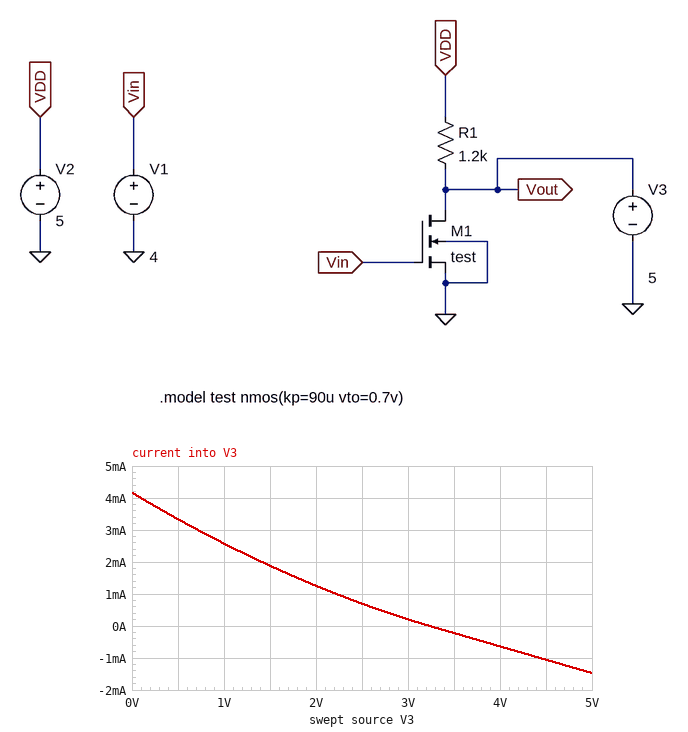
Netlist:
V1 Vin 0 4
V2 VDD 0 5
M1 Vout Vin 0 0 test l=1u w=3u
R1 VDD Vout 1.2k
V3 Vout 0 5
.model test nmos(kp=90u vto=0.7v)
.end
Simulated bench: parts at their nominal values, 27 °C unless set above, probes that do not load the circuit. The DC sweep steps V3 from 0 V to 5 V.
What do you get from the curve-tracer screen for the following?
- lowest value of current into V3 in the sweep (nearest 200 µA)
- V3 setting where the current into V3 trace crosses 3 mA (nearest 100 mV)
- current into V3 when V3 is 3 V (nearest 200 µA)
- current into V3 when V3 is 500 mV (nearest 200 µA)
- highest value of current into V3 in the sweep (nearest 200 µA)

-1.4 mA
700 mV
200 µA
3.4 mA
4.2 mA
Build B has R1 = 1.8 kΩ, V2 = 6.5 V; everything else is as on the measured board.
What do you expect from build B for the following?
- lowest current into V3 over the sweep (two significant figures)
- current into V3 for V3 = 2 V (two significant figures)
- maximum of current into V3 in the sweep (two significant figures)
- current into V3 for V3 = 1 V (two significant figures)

-640 µA
1.3 mA
3.6 mA
2.3 mA
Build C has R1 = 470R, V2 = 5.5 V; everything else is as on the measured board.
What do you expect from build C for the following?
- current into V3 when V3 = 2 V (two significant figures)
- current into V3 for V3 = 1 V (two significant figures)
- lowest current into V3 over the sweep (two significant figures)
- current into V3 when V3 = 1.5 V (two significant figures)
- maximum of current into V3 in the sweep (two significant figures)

6.2 mA
8.8 mA
-410 µA
7.5 mA
12 mA
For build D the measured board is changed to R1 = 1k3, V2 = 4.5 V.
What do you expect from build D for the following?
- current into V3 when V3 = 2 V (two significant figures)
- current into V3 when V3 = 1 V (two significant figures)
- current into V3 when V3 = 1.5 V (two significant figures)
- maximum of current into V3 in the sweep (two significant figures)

680 µA
1.9 mA
1.3 mA
3.5 mA
